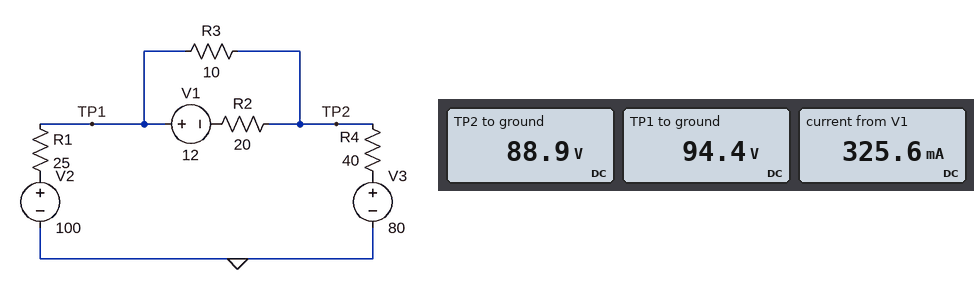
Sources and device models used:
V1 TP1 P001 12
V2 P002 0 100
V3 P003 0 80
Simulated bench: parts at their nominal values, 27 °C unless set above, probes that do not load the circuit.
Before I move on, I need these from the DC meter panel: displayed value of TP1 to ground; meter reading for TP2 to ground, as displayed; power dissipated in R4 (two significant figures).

94.4 V
88.9 V
2.0 W
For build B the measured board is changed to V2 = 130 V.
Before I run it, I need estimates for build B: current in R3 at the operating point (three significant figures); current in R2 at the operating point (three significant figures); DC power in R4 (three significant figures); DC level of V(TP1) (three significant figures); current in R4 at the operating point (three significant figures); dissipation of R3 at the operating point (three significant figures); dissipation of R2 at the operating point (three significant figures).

828 mA
186 mA
16.5 W
114 V
642 mA
6.85 W
692 mW
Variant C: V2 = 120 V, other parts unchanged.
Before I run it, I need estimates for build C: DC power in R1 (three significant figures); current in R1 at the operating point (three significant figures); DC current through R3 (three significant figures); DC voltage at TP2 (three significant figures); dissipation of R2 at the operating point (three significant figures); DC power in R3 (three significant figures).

6.31 W
502 mA
735 mA
100 V
1.08 W
5.40 W
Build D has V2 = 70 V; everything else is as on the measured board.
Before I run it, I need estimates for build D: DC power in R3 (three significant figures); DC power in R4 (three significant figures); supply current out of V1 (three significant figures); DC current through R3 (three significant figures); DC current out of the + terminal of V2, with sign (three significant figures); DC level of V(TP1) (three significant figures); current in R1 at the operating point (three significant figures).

728 mW
1.53 W
465 mA
270 mA
-195 mA
74.9 V
195 mA
